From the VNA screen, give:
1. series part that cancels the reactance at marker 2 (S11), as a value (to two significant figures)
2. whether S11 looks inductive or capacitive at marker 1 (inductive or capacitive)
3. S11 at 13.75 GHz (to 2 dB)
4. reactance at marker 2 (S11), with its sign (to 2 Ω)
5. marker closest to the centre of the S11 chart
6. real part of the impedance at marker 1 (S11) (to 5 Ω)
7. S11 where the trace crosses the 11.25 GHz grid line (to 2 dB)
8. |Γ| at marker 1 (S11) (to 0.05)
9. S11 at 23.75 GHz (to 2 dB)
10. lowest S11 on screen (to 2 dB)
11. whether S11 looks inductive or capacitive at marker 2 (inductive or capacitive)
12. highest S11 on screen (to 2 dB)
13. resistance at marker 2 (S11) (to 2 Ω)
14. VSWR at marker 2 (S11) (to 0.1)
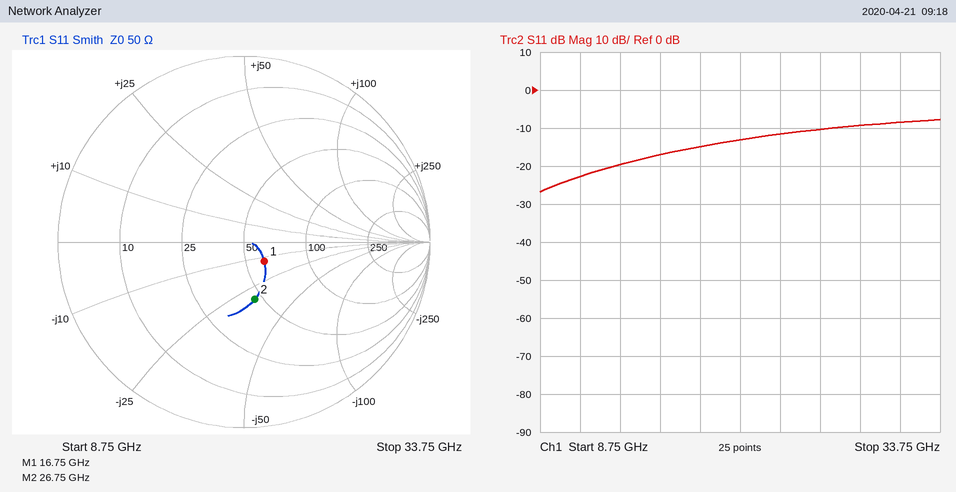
190 pH
capacitive
-20 dB
-32 Ω
marker 1
60 Ω
-22 dB
0.15
-12 dB
-26 dB
capacitive
-8 dB
46 Ω
1.9
